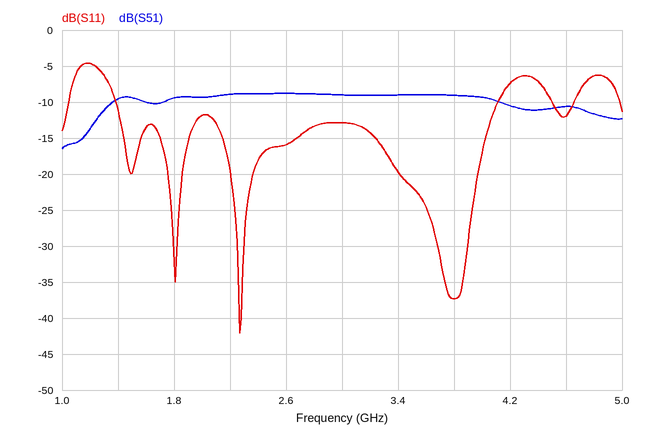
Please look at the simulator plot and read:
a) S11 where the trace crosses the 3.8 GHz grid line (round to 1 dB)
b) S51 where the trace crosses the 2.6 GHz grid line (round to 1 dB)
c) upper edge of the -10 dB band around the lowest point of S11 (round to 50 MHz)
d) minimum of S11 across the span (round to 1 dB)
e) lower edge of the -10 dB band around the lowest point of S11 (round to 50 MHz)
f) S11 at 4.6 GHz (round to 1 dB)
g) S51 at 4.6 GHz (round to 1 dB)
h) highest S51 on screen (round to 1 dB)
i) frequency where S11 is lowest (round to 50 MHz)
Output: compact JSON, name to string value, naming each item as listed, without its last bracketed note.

{"S11 where the trace crosses the 3.8 GHz grid line": "-37 dB", "S51 where the trace crosses the 2.6 GHz grid line": "-9 dB", "upper edge of the -10 dB band around the lowest point of S11": "4.10 GHz", "minimum of S11 across the span": "-42 dB", "lower edge of the -10 dB band around the lowest point of S11": "1.40 GHz", "S11 at 4.6 GHz": "-12 dB", "S51 at 4.6 GHz": "-11 dB", "highest S51 on screen": "-9 dB", "frequency where S11 is lowest": "2.25 GHz"}
